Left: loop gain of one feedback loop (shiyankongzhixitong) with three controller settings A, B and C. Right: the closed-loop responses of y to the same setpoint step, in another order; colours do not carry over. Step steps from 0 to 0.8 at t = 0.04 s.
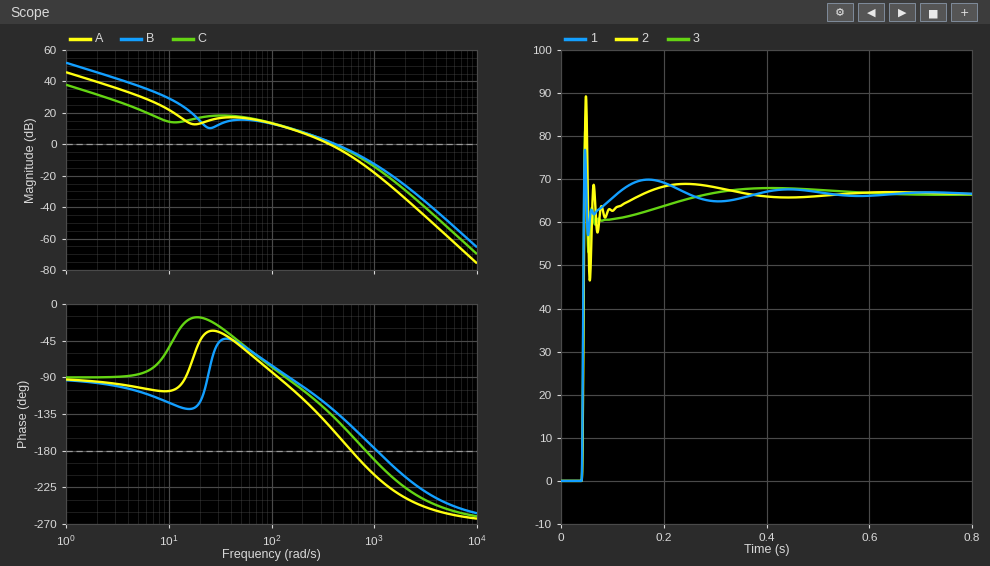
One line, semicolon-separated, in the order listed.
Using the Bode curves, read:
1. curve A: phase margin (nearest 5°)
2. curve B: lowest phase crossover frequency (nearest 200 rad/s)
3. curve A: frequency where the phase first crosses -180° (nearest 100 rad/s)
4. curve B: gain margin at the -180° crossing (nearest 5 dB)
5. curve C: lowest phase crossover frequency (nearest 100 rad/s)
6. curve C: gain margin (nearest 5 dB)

30°; 1000 rad/s; 600 rad/s; 15 dB; 800 rad/s; 10 dB
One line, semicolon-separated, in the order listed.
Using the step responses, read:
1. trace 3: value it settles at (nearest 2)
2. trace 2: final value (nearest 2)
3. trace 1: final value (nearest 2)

66; 66; 66
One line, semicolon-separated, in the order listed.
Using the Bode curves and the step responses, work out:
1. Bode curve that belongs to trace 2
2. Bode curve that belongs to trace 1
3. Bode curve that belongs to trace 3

A; B; C
